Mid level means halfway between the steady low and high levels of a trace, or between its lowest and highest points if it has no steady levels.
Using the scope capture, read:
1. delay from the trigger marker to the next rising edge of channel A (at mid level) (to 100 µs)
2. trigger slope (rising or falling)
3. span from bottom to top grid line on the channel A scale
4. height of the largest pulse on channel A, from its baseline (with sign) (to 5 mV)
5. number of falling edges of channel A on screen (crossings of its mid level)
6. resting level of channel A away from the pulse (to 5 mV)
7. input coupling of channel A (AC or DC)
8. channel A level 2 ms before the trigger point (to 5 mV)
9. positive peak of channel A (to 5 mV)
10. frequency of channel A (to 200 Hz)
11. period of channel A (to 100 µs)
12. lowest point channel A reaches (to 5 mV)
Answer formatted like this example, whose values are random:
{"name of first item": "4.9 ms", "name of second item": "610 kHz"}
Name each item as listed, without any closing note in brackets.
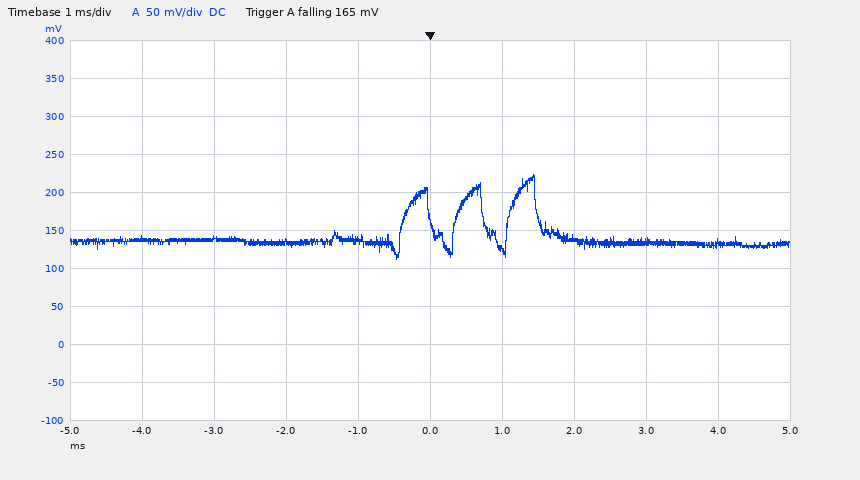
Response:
{"delay from the trigger marker to the next rising edge of channel A (at mid level)": "400 µs", "trigger slope": "falling", "span from bottom to top grid line on the channel A scale": "500 mV", "height of the largest pulse on channel A, from its baseline (with sign)": "+90 mV", "number of falling edges of channel A on screen": "3", "resting level of channel A away from the pulse": "135 mV", "input coupling of channel A": "DC", "channel A level 2 ms before the trigger point": "135 mV", "positive peak of channel A": "225 mV", "frequency of channel A": "1.4 kHz", "period of channel A": "700 µs", "lowest point channel A reaches": "110 mV"}
